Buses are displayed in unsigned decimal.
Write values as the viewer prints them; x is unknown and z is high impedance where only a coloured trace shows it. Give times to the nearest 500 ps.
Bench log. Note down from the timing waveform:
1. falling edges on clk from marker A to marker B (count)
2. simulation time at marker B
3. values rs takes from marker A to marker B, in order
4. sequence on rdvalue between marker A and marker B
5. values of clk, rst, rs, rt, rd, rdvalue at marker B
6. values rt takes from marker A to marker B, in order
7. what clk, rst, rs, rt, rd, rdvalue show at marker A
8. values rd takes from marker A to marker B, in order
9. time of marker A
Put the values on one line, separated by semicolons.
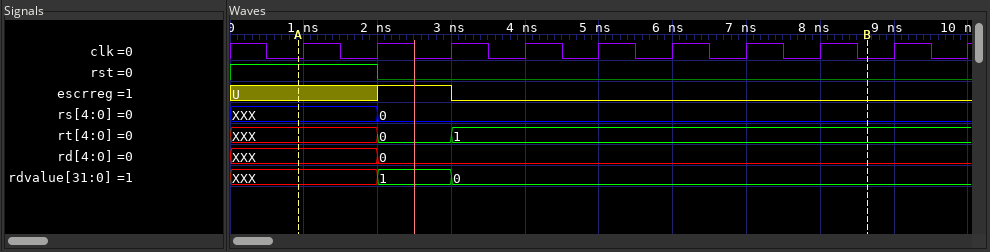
8; 8500 ps; XXX, 0; XXX, 1, 0; clk=0, rst=0, rs=0, rt=1, rd=0, rdvalue=0; XXX, 0, 1; clk=0, rst=1, rs=XXX, rt=XXX, rd=XXX, rdvalue=XXX; XXX, 0; 1000 ps
